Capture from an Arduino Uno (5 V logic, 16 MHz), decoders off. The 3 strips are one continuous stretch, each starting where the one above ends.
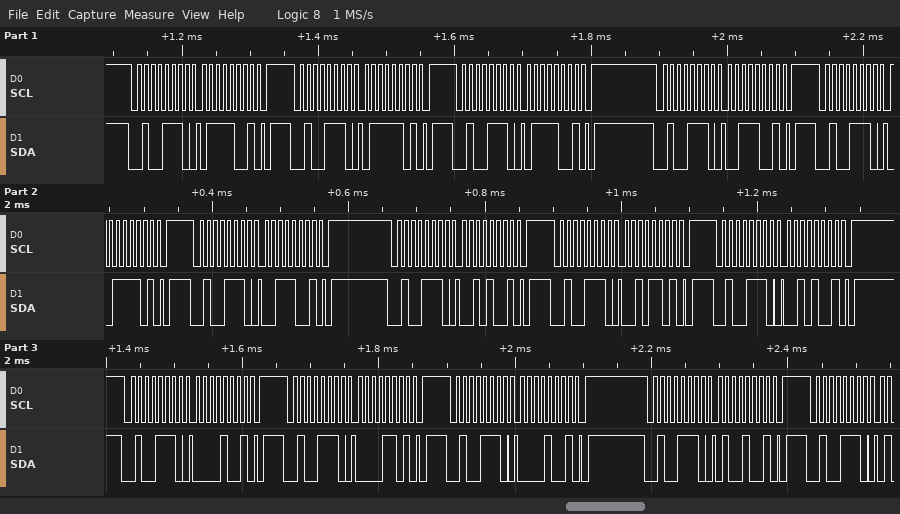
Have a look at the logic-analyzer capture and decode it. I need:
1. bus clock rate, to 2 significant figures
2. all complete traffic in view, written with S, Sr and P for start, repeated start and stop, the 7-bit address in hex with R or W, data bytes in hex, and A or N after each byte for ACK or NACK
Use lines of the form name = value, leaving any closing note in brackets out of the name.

bus clock rate, to 2 significant figures = 100 kHz
all complete traffic in view, written with S, Sr and P for start, repeated start and stop, the 7-bit address in hex with R or W, data bytes in hex, and A or N after each byte for ACK or NACK = S 27W A 79 A P S 27W A 7D A P S 27W A 79 A P S 27W A 39 A P S 27W A 3D A P S 27W A 39 A P S 27W A 29 A P S 27W A 2D A P S 27W A 29 A P S 27W A 09 A P S 27W A 0D A P S 27W A 09 A P S 27W A 49 A P S 27W A
